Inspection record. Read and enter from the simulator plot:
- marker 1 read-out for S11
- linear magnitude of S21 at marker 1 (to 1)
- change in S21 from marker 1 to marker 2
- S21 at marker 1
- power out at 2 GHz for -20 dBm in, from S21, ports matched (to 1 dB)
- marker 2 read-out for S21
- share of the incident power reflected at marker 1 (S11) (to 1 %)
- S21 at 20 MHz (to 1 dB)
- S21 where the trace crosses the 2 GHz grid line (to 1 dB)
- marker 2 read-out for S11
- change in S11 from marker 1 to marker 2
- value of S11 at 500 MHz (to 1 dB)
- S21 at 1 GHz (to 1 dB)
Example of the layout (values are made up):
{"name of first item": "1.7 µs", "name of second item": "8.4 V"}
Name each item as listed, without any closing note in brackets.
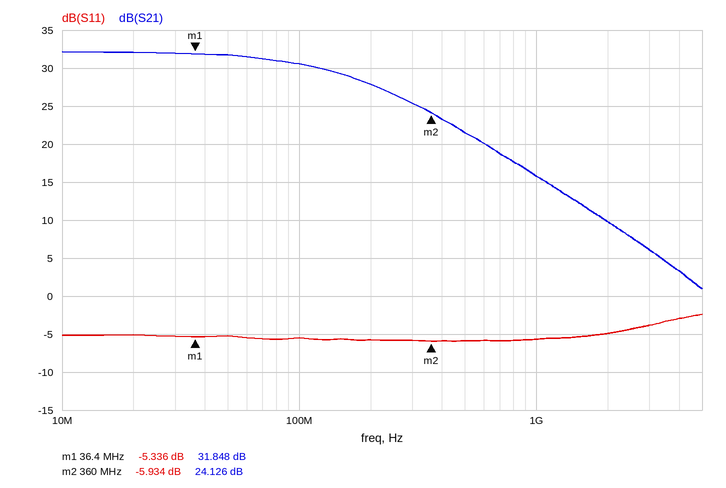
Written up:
{"marker 1 read-out for S11": "-5.336 dB", "linear magnitude of S21 at marker 1": "39", "change in S21 from marker 1 to marker 2": "-7.722 dB", "S21 at marker 1": "31.848 dB", "power out at 2 GHz for -20 dBm in, from S21, ports matched": "-10 dBm", "marker 2 read-out for S21": "24.126 dB", "share of the incident power reflected at marker 1 (S11)": "29 %", "S21 at 20 MHz": "32 dB", "S21 where the trace crosses the 2 GHz grid line": "10 dB", "marker 2 read-out for S11": "-5.934 dB", "change in S11 from marker 1 to marker 2": "-0.598 dB", "value of S11 at 500 MHz": "-6 dB", "S21 at 1 GHz": "16 dB"}
